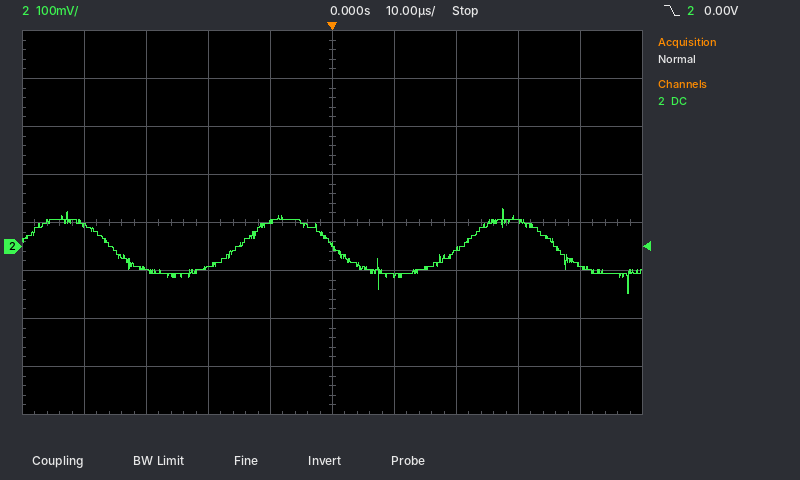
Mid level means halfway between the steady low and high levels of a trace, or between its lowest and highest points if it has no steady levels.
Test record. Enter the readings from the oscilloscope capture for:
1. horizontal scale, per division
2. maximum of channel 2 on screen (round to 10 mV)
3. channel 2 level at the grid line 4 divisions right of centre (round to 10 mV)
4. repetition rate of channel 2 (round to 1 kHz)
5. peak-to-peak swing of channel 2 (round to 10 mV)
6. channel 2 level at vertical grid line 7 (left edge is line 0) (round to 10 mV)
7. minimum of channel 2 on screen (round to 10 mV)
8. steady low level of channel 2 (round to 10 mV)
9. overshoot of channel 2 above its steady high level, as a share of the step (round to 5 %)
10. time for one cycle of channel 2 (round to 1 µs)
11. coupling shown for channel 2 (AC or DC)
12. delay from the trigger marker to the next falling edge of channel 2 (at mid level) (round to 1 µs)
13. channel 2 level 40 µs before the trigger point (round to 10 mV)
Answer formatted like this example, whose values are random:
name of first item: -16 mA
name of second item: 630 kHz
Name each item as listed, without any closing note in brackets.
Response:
horizontal scale, per division: 10 µs
maximum of channel 2 on screen: 80 mV
channel 2 level at the grid line 4 divisions right of centre: -40 mV
repetition rate of channel 2: 28 kHz
peak-to-peak swing of channel 2: 180 mV
channel 2 level at vertical grid line 7 (left edge is line 0): -10 mV
minimum of channel 2 on screen: -100 mV
steady low level of channel 2: -60 mV
overshoot of channel 2 above its steady high level, as a share of the step: 20 %
time for one cycle of channel 2: 36 µs
coupling shown for channel 2: DC
delay from the trigger marker to the next falling edge of channel 2 (at mid level): 36 µs
channel 2 level 40 µs before the trigger point: 40 mV
